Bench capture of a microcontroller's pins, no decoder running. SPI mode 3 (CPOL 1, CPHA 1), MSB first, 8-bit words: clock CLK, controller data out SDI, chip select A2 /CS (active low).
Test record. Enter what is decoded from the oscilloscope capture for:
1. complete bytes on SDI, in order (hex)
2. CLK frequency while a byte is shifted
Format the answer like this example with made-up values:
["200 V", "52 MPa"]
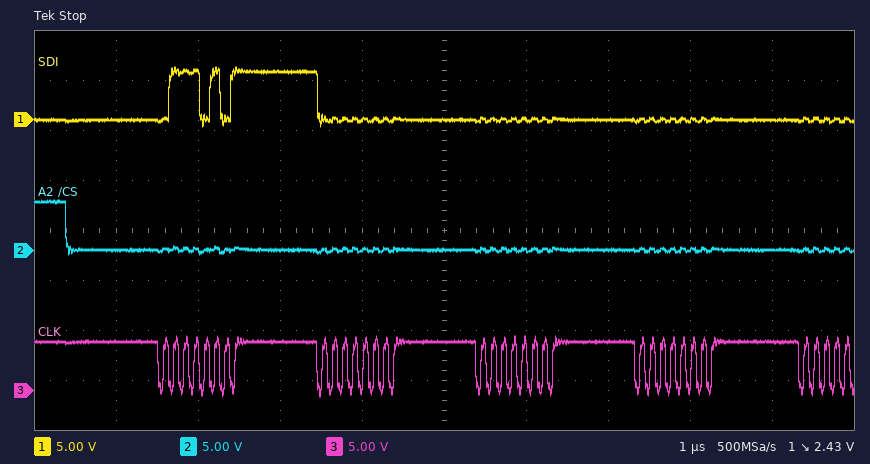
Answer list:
["0x75 0x00 0x00 0x00", "8 MHz"]
